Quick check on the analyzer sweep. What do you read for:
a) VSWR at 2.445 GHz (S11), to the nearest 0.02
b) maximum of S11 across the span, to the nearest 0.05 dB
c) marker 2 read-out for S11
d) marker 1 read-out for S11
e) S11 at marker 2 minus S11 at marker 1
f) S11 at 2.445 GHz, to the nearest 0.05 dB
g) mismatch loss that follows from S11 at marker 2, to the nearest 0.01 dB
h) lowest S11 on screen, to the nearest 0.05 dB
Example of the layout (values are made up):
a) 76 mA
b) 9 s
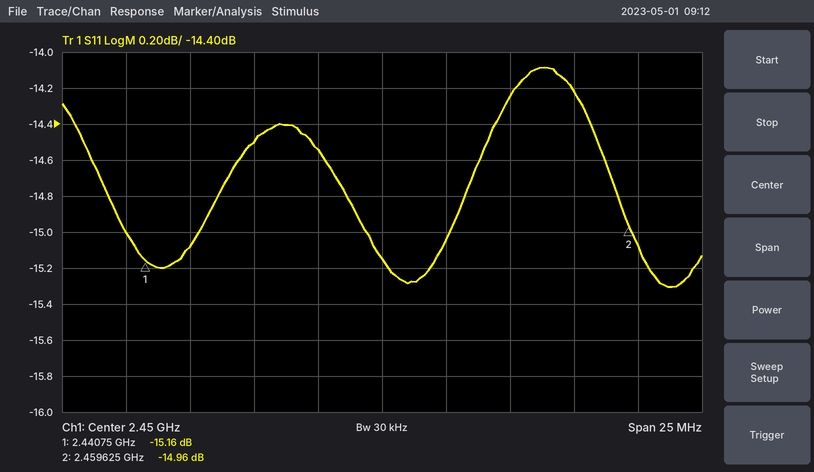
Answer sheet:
a) 1.46
b) -14.10 dB
c) -14.96 dB
d) -15.16 dB
e) 0.20 dB
f) -14.50 dB
g) 0.14 dB
h) -15.30 dB
